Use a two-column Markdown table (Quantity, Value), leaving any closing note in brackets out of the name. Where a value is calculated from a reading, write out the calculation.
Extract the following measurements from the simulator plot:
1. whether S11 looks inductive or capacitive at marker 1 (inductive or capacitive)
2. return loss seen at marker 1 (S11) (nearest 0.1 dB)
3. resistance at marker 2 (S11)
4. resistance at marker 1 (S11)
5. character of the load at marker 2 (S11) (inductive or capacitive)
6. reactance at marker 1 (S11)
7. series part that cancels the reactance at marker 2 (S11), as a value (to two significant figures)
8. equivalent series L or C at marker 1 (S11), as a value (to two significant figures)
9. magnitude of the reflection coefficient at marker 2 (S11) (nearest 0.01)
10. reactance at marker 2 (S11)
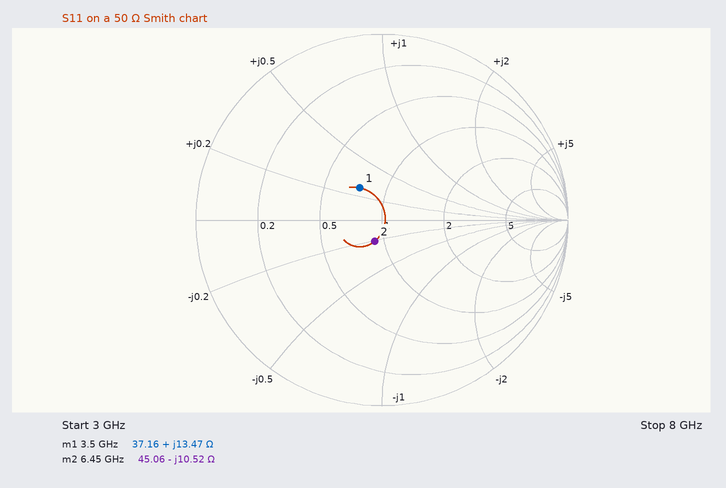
| Quantity | Value |
|---|---|
| whether S11 looks inductive or capacitive at marker 1 | inductive |
| return loss seen at marker 1 (S11) | 13.5 dB |
| resistance at marker 2 | 45.06 Ω |
| resistance at marker 1 | 37.16 Ω |
| character of the load at marker 2 (S11) | capacitive |
| reactance at marker 1 | +13.47 Ω |
| series part that cancels the reactance at marker 2 (S11), as a value | L = 10.52 Ω/(2π × 6.45 GHz) ≈ 260 pH |
| equivalent series L or C at marker 1 (S11), as a value | L = 13.47 Ω/(2π × 3.5 GHz) ≈ 613 pH, so 610 pH to two significant figures |
| magnitude of the reflection coefficient at marker 2 (S11) | 0.12 |
| reactance at marker 2 | -10.52 Ω |
